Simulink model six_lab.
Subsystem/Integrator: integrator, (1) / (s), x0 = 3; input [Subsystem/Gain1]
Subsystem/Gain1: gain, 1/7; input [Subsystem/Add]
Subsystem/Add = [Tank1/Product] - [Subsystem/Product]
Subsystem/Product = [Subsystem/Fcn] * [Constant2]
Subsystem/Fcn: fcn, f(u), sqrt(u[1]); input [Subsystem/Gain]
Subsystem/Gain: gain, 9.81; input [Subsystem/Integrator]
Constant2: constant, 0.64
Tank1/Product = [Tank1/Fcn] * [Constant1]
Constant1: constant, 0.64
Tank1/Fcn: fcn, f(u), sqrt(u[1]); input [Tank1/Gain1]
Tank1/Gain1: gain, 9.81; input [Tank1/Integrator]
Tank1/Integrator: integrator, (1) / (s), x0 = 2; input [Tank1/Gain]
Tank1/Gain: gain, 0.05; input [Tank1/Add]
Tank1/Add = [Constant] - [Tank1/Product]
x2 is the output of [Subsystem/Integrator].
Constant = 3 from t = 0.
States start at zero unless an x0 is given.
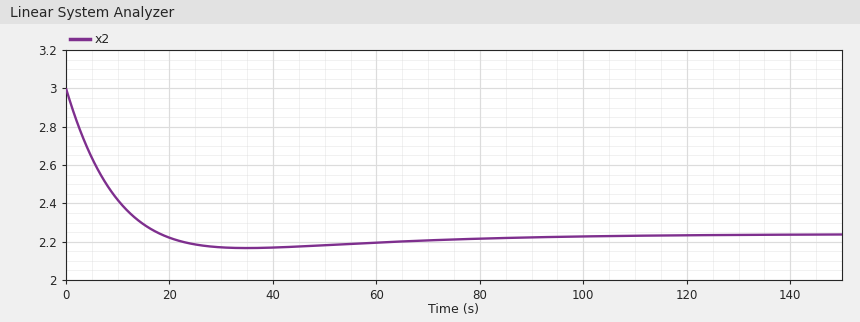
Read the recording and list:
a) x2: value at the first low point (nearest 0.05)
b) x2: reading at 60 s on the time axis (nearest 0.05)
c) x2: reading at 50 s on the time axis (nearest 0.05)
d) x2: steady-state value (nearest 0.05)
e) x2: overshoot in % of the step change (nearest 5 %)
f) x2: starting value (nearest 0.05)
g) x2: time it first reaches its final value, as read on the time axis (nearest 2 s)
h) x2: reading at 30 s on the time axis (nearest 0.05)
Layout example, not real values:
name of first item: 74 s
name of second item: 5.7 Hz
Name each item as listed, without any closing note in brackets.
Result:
x2: value at the first low point: 2.15
x2: reading at 60 s on the time axis: 2.20
x2: reading at 50 s on the time axis: 2.20
x2: steady-state value: 2.25
x2: overshoot in % of the step change: 10 %
x2: starting value: 3.00
x2: time it first reaches its final value, as read on the time axis: 18 s
x2: reading at 30 s on the time axis: 2.15
